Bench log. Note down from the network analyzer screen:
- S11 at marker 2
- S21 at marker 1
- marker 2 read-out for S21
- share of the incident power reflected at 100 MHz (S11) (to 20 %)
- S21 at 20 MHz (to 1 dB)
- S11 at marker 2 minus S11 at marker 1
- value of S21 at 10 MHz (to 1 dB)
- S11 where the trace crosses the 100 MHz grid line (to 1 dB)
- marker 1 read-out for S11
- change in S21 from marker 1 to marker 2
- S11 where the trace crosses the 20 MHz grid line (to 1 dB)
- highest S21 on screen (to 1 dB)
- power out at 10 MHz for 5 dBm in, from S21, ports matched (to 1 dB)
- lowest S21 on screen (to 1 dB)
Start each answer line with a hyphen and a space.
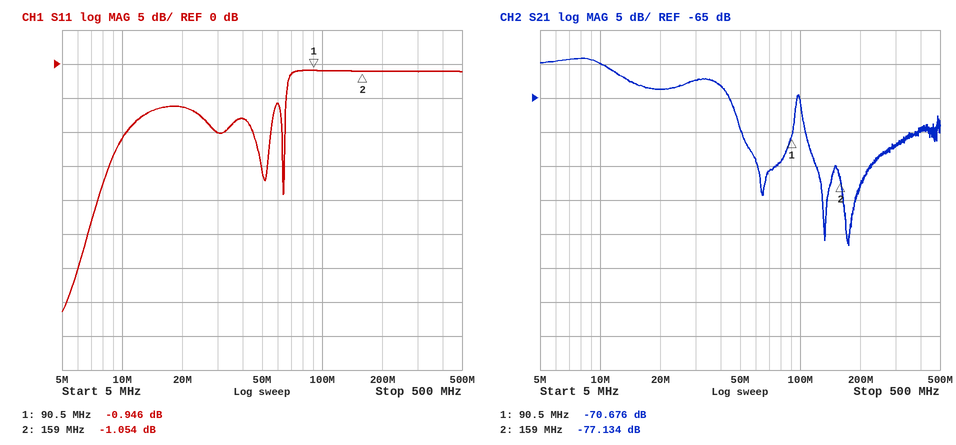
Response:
- -1.054 dB
- -70.676 dB
- -77.134 dB
- 80 %
- -64 dB
- -0.108 dB
- -60 dB
- -1 dB
- -0.946 dB
- -6.458 dB
- -6 dB
- -59 dB
- -55 dBm
- -87 dB
